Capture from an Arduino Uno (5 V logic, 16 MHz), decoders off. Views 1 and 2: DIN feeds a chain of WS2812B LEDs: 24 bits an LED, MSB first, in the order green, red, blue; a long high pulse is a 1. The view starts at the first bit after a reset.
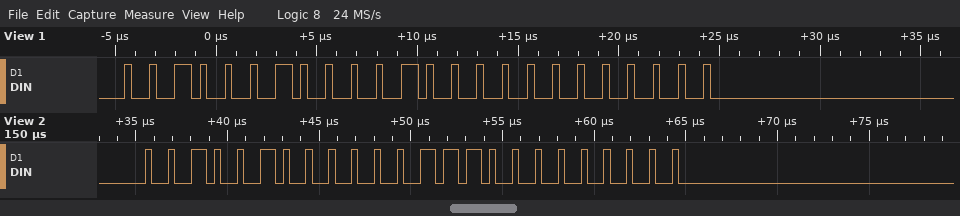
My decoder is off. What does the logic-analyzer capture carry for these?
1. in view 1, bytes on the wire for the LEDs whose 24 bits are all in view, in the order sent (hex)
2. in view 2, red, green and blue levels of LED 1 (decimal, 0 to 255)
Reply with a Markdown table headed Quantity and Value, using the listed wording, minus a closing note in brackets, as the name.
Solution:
| Quantity | Value |
|---|---|
| in view 1, bytes on the wire for the LEDs whose 24 bits are all in view, in the order sent | 22 10 00 |
| in view 2, red, green and blue levels of LED 1 | 14, 36, 0 |
